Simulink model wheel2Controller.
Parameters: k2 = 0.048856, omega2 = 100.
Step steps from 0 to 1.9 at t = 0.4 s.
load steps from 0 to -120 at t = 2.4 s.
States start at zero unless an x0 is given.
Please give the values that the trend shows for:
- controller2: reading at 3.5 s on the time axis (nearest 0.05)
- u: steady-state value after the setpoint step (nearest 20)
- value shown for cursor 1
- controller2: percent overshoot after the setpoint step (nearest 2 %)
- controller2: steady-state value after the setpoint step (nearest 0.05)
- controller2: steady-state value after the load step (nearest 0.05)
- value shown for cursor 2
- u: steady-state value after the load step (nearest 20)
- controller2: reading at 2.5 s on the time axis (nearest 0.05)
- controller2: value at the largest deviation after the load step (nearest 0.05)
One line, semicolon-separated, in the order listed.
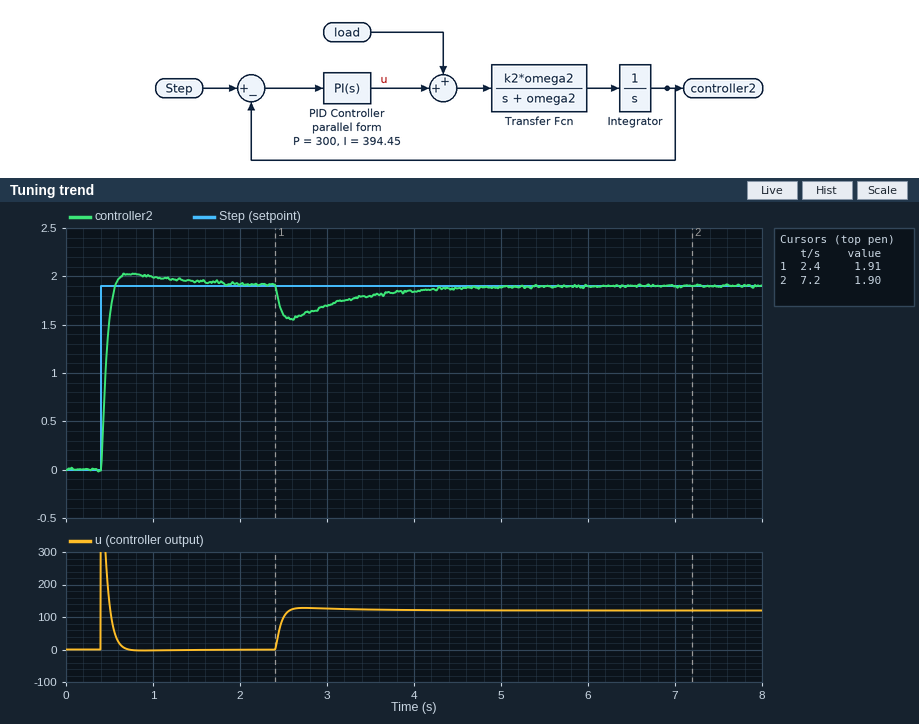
1.80; 0; 1.91; 6 %; 1.90; 1.90; 1.90; 120; 1.60; 1.55
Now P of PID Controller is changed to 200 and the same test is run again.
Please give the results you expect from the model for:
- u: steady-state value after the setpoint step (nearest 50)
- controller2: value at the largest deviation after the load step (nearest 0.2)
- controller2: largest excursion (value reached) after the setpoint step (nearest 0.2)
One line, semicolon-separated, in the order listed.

0; 1.4; 2.2
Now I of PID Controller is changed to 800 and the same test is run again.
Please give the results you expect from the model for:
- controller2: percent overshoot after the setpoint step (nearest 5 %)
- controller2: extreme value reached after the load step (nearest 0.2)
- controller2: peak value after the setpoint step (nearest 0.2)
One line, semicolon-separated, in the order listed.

10 %; 1.6; 2.2
